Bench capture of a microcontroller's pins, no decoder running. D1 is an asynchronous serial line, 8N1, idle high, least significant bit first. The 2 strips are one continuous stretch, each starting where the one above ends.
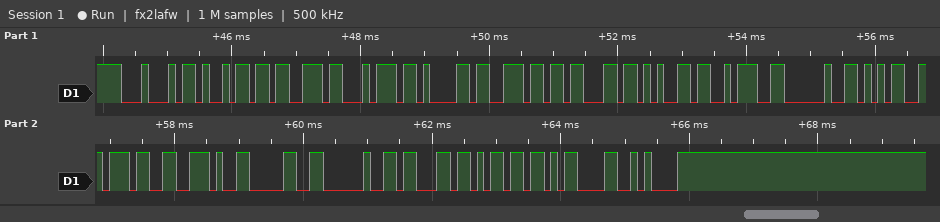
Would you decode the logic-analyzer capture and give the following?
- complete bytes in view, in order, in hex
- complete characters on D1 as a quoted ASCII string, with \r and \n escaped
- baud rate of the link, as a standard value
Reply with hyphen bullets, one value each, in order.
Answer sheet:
- 44 69 73 74 61 6E 63 65 3A 20 35 37 2E 30 20 63 6D 0D 0A
- "Distance: 57.0 cm\r\n"
- 9600 baud
